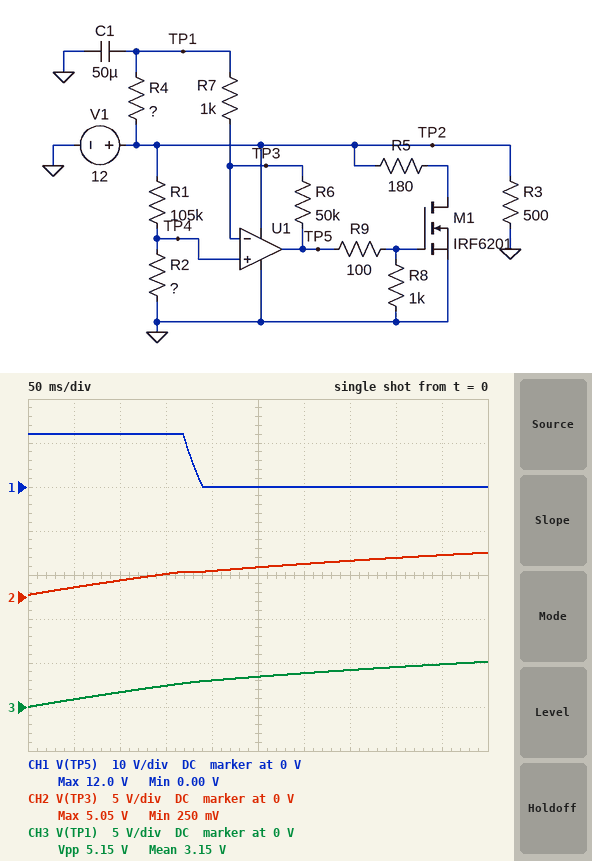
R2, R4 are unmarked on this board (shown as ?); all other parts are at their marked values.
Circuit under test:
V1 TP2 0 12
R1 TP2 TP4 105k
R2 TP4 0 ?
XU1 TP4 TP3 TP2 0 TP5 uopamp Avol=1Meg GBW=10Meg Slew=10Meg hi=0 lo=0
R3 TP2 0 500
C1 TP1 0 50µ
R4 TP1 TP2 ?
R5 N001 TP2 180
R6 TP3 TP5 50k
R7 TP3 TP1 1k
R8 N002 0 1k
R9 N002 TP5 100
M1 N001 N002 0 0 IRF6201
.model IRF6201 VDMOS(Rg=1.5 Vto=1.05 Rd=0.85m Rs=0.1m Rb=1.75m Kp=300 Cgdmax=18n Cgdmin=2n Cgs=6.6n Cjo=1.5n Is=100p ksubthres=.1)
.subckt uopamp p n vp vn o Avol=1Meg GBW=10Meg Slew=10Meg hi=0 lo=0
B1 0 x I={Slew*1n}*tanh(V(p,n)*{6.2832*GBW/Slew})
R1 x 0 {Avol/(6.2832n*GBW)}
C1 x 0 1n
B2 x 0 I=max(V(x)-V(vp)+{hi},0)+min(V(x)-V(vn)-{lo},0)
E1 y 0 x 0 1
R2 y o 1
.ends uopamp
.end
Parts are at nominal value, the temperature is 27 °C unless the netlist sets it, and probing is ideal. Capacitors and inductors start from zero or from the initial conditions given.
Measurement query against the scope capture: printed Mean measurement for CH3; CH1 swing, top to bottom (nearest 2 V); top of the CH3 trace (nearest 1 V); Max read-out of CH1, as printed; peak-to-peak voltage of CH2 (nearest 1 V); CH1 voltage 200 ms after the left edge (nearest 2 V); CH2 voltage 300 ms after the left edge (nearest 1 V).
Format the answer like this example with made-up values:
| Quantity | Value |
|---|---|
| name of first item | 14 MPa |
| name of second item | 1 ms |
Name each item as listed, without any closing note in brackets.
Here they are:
| Quantity | Value |
|---|---|
| printed Mean measurement for CH3 | 3.15 V |
| CH1 swing, top to bottom | 12 V |
| top of the CH3 trace | 5 V |
| Max read-out of CH1, as printed | 12.0 V |
| peak-to-peak voltage of CH2 | 5 V |
| CH1 voltage 200 ms after the left edge | 0 V |
| CH2 voltage 300 ms after the left edge | 4 V |
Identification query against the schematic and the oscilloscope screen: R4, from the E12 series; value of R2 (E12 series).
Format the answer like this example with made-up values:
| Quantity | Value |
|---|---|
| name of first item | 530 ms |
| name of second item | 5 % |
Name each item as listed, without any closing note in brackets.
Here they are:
| Quantity | Value |
|---|---|
| R4, from the E12 series | 18 kΩ |
| value of R2 | 33 kΩ |
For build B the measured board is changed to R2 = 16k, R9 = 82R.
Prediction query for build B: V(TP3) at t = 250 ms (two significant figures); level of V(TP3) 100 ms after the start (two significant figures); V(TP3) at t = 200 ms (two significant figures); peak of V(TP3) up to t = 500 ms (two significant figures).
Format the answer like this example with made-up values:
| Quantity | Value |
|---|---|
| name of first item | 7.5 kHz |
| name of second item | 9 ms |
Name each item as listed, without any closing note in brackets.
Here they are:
| Quantity | Value |
|---|---|
| V(TP3) at t = 250 ms | 3.0 V |
| level of V(TP3) 100 ms after the start | 1.6 V |
| V(TP3) at t = 200 ms | 2.6 V |
| peak of V(TP3) up to t = 500 ms | 4.8 V |
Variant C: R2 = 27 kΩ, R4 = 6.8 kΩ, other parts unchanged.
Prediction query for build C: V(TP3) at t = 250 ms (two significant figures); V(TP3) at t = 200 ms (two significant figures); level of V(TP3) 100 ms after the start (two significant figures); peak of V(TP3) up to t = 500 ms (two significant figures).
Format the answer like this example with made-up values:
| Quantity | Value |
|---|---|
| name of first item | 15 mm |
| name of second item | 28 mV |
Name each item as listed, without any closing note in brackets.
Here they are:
| Quantity | Value |
|---|---|
| V(TP3) at t = 250 ms | 6.0 V |
| V(TP3) at t = 200 ms | 5.2 V |
| level of V(TP3) 100 ms after the start | 3.2 V |
| peak of V(TP3) up to t = 500 ms | 8.5 V |
